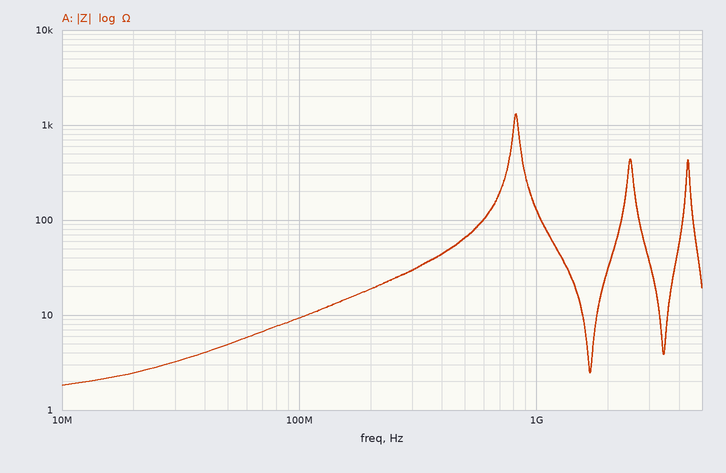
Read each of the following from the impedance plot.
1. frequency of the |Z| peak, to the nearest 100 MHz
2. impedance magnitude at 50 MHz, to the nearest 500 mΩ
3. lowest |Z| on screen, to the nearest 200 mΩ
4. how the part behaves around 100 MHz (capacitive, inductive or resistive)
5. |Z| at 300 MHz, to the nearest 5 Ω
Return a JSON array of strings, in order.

["800 MHz", "5.0 Ω", "1.8 Ω", "inductive", "30 Ω"]
